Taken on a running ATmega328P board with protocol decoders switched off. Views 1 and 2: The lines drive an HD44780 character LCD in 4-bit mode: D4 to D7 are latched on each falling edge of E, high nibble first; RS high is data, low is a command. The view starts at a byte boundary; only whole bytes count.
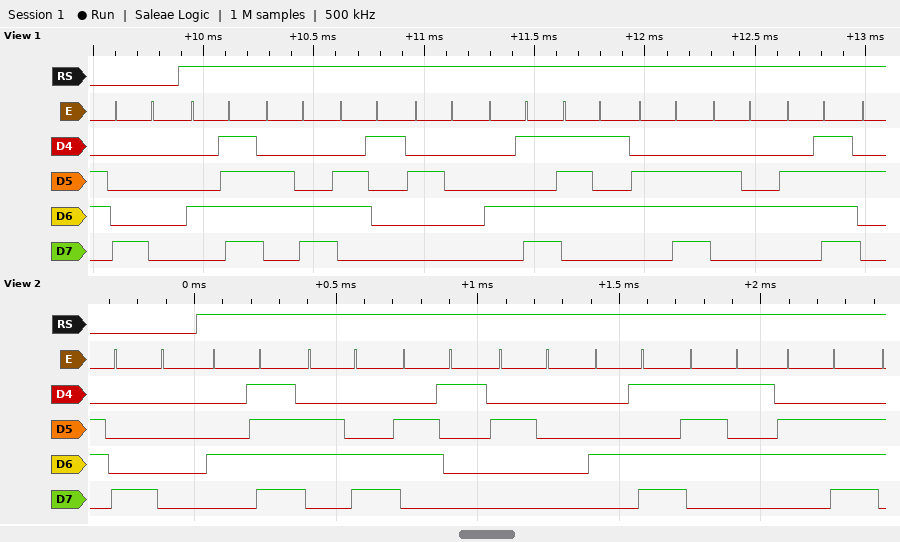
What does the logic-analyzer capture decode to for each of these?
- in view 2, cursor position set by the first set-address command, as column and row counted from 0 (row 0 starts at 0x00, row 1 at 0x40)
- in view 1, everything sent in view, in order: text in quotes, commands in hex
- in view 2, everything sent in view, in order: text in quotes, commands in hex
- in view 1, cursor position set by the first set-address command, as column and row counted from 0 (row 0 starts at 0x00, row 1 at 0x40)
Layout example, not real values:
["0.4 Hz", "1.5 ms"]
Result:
["column 0, row 0", "0x80 \"Ola Mundo\"", "0x80 \"Ola Mun\"", "column 0, row 0"]
